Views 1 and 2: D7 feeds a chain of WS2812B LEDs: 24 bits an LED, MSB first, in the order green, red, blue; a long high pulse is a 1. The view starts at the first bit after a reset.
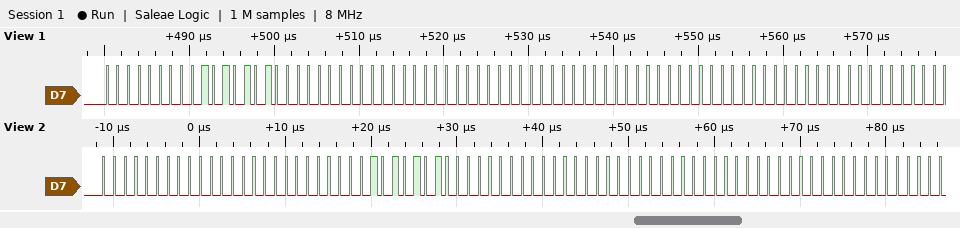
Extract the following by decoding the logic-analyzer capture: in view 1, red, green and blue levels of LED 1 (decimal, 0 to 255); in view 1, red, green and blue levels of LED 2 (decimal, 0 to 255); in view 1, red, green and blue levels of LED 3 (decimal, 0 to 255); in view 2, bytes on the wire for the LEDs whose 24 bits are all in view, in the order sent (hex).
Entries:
85, 0, 0
0, 0, 0
0, 0, 0
00 00 00 55 00 00 00 00 00
